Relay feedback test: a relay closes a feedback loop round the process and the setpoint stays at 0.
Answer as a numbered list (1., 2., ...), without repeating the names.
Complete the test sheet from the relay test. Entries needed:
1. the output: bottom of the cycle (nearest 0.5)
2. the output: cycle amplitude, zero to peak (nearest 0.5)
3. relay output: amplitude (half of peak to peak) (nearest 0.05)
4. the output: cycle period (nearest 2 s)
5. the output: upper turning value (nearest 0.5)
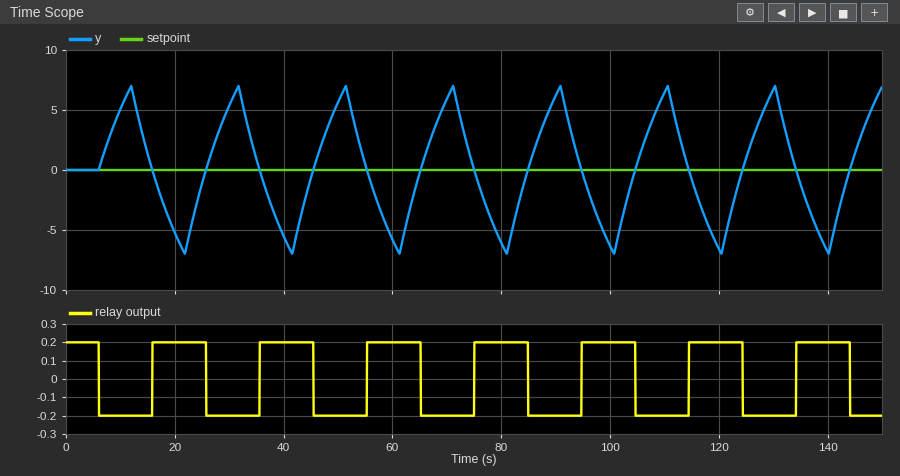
1. -7.0
2. 7.0
3. 0.20
4. 20 s
5. 7.0
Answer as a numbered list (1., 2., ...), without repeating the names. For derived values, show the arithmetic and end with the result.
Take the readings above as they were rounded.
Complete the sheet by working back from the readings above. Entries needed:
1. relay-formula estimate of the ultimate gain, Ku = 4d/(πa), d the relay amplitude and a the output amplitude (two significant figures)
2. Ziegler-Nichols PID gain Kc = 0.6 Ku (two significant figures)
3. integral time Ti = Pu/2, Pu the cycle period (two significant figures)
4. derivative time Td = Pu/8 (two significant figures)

1. 4 × 0.2 / (π × 7) = 0.036
2. 0.6 × 0.036 = 0.022
3. 20 / 2 = 10 s
4. 20 / 8 = 2.5 s
